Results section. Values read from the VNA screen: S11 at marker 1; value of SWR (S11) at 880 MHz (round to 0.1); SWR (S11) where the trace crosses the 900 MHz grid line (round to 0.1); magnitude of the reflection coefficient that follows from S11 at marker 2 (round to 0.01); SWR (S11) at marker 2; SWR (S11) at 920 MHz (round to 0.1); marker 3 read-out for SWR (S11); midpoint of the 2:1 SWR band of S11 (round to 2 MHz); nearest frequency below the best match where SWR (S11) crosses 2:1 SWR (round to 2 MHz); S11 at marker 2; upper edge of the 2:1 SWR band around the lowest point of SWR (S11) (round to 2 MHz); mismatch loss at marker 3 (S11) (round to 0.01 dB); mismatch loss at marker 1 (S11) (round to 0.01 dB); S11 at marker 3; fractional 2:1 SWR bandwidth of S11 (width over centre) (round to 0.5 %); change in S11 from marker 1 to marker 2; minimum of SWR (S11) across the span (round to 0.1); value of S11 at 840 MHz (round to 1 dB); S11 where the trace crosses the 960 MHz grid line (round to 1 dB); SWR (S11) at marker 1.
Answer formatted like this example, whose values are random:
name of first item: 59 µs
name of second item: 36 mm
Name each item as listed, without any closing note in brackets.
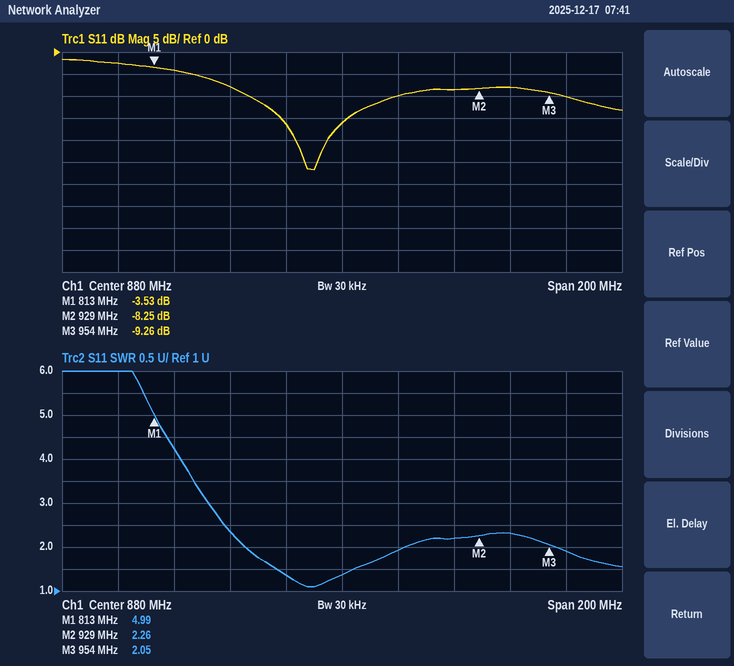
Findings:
S11 at marker 1: -3.53 dB
value of SWR (S11) at 880 MHz: 1.4
SWR (S11) where the trace crosses the 900 MHz grid line: 1.9
magnitude of the reflection coefficient that follows from S11 at marker 2: 0.39
SWR (S11) at marker 2: 2.26
SWR (S11) at 920 MHz: 2.2
marker 3 read-out for SWR: 2.05
midpoint of the 2:1 SWR band of S11: 874 MHz
nearest frequency below the best match where SWR (S11) crosses 2:1 SWR: 846 MHz
S11 at marker 2: -8.25 dB
upper edge of the 2:1 SWR band around the lowest point of SWR (S11): 902 MHz
mismatch loss at marker 3 (S11): 0.55 dB
mismatch loss at marker 1 (S11): 2.55 dB
S11 at marker 3: -9.26 dB
fractional 2:1 SWR bandwidth of S11 (width over centre): 6.5 %
change in S11 from marker 1 to marker 2: -4.72 dB
minimum of SWR (S11) across the span: 1.1
value of S11 at 840 MHz: -8 dB
S11 where the trace crosses the 960 MHz grid line: -10 dB
SWR (S11) at marker 1: 4.99
